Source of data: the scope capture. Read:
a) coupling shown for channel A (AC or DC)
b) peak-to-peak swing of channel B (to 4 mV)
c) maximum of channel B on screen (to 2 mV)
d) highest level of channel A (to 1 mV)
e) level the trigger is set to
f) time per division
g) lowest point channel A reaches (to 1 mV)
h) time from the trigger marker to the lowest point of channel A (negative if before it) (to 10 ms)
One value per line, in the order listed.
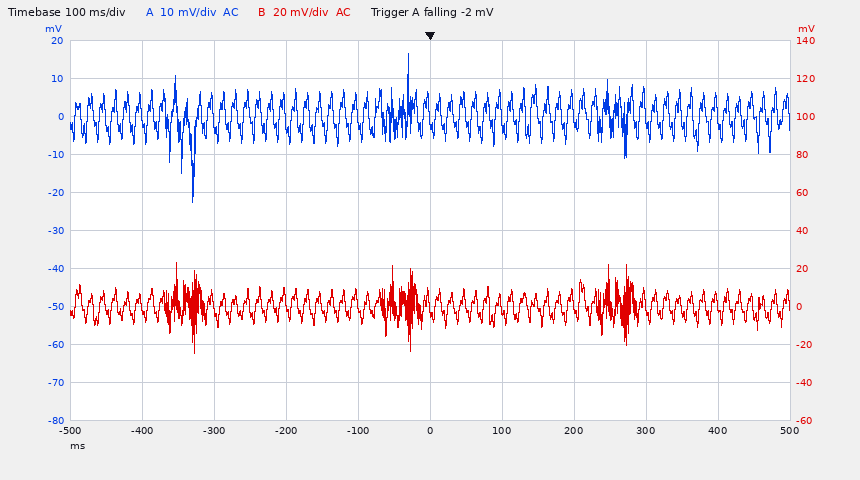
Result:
AC
48 mV
24 mV
17 mV
-2 mV
100 ms
-23 mV
-330 ms
